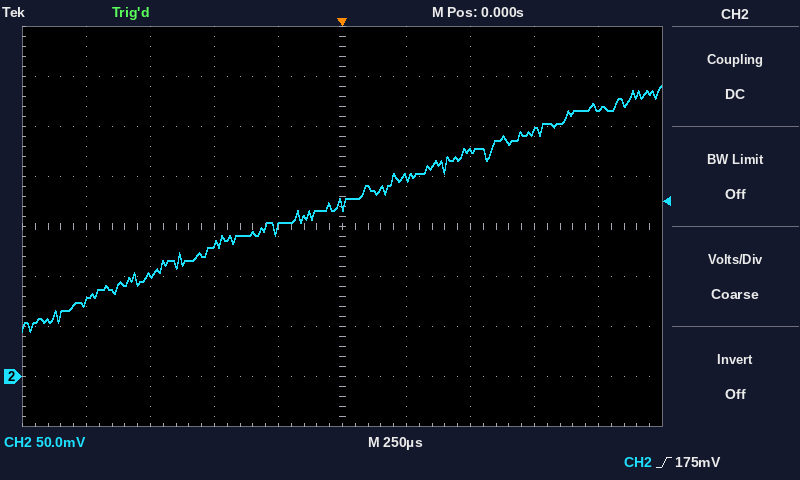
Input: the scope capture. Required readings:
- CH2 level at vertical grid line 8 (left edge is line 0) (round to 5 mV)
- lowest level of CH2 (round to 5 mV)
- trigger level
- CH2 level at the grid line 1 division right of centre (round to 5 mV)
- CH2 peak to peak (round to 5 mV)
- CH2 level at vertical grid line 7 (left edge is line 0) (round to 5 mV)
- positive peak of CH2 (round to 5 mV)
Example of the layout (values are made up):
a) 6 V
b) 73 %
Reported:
a) 245 mV
b) 45 mV
c) 175 mV
d) 200 mV
e) 245 mV
f) 225 mV
g) 290 mV
